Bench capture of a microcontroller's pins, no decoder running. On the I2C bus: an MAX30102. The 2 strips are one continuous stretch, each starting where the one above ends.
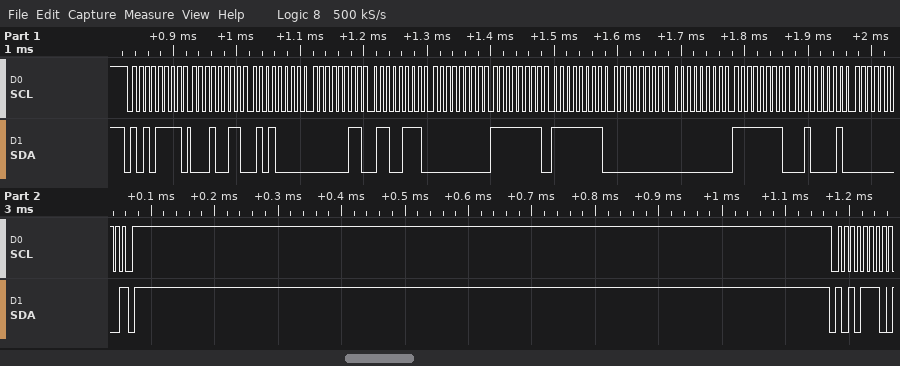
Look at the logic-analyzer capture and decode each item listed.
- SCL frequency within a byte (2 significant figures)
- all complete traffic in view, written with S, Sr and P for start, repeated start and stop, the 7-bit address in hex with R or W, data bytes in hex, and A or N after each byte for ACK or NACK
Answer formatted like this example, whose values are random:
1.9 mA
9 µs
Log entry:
100 kHz
S 57R A 13 A 50 A 03 A 67 A 00 A FF A FF A 00 A 00 A FF A 21 A 00 N P S 57W A
